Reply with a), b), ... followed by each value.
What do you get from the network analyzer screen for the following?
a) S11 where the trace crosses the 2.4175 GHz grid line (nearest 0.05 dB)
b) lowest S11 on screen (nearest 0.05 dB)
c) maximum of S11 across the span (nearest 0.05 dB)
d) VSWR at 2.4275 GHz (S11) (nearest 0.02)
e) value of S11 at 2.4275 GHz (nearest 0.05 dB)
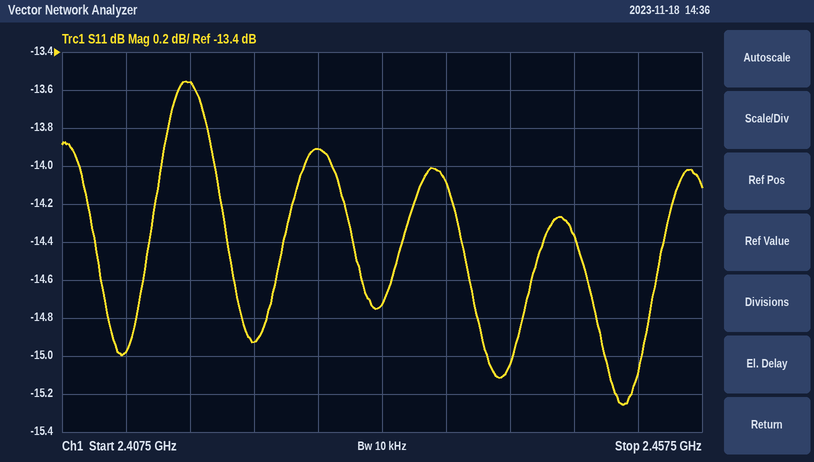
a) -13.55 dB
b) -15.25 dB
c) -13.55 dB
d) 1.50
e) -13.90 dB
